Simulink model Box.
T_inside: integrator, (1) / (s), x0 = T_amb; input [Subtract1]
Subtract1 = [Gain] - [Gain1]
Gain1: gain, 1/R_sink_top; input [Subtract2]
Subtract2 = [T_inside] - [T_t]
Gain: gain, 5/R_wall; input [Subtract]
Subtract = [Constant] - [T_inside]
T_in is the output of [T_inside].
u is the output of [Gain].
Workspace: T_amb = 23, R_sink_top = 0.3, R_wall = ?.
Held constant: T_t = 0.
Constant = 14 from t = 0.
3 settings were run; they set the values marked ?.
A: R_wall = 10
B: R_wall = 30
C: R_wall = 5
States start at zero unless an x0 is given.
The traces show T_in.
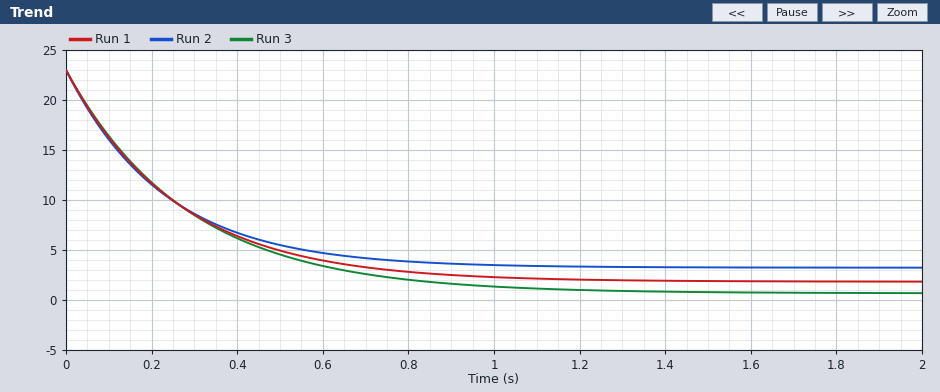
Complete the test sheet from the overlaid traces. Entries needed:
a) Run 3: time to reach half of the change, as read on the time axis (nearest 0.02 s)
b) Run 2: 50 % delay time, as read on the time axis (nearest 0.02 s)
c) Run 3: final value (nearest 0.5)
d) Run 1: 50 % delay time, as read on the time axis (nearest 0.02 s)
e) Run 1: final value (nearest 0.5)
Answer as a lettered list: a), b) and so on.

a) 0.20 s
b) 0.16 s
c) 0.5
d) 0.18 s
e) 2.0
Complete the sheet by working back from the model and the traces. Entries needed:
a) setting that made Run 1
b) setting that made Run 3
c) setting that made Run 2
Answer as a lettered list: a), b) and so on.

a) A
b) B
c) C
